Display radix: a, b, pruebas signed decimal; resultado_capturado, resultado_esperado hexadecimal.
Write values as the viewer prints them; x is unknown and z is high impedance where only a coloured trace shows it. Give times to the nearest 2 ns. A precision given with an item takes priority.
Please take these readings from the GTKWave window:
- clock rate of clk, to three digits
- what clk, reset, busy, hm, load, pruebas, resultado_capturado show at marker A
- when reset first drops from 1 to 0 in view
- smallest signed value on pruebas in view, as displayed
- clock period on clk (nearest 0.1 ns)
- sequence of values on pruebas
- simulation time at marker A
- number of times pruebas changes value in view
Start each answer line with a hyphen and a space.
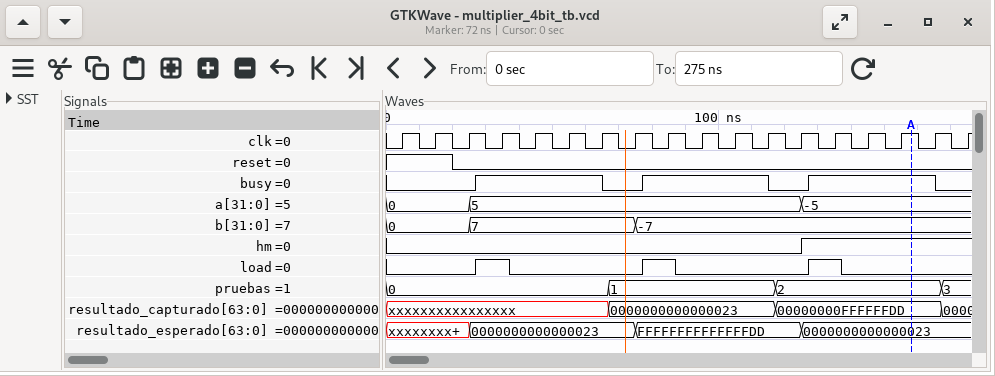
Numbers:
- 100 MHz
- clk=1, reset=0, busy=1, hm=1, load=0, pruebas=2, resultado_capturado=00000000FFFFFFDD
- 20 ns
- 0
- 10 ns
- 0, 1, 2, 3
- 158 ns
- 3
